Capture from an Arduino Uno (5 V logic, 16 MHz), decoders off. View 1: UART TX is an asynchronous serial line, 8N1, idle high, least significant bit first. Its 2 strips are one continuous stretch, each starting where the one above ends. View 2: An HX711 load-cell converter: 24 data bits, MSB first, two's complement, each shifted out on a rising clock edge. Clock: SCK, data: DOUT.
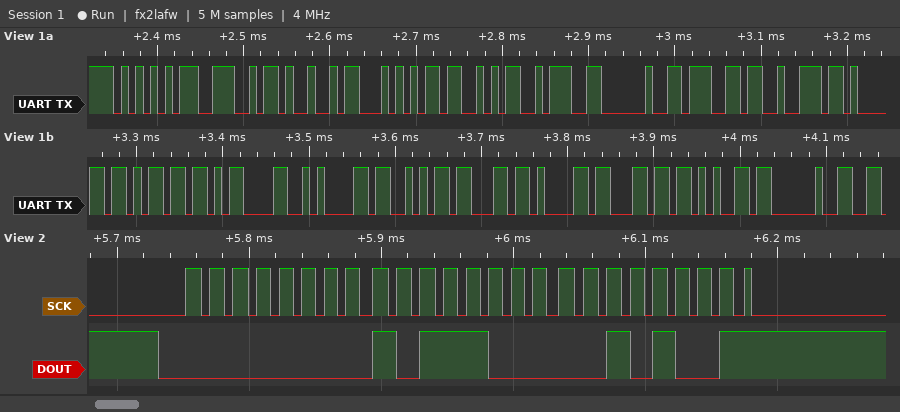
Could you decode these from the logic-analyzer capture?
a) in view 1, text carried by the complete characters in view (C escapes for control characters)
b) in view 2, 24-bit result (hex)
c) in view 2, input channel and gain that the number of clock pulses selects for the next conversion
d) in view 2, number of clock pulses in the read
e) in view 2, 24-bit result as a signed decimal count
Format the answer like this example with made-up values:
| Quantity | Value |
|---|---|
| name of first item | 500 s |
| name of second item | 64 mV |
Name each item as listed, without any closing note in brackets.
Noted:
| Quantity | Value |
|---|---|
| in view 1, text carried by the complete characters in view | "UNITS: gram\r\nScale " |
| in view 2, 24-bit result | 0x00B829 |
| in view 2, input channel and gain that the number of clock pulses selects for the next conversion | channel A, gain 128 |
| in view 2, number of clock pulses in the read | 25 |
| in view 2, 24-bit result as a signed decimal count | 47145 |
